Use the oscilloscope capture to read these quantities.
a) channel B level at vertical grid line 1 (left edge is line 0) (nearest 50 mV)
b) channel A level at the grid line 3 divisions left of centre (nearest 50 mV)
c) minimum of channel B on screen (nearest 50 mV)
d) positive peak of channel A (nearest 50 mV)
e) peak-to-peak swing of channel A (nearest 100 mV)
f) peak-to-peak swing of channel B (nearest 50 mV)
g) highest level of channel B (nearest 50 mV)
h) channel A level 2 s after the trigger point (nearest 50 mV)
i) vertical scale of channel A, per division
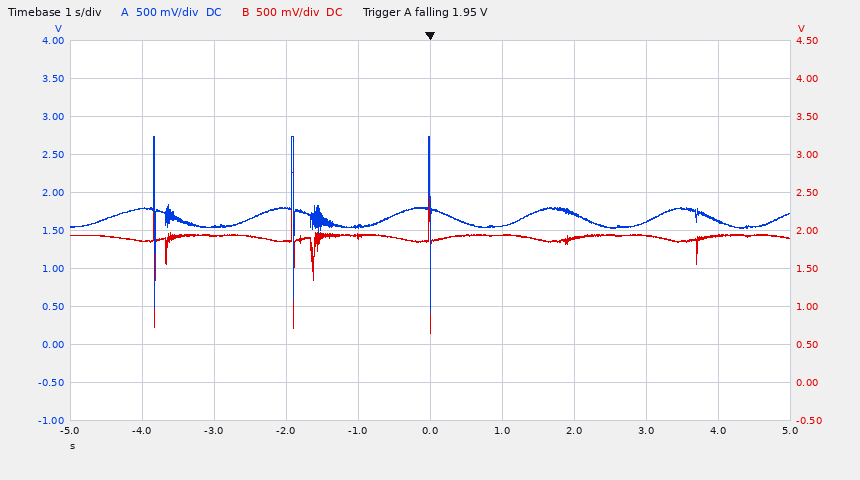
1.85 V
1.55 V
650 mV
2.75 V
2.30 V
2.10 V
2.75 V
1.70 V
500 mV
